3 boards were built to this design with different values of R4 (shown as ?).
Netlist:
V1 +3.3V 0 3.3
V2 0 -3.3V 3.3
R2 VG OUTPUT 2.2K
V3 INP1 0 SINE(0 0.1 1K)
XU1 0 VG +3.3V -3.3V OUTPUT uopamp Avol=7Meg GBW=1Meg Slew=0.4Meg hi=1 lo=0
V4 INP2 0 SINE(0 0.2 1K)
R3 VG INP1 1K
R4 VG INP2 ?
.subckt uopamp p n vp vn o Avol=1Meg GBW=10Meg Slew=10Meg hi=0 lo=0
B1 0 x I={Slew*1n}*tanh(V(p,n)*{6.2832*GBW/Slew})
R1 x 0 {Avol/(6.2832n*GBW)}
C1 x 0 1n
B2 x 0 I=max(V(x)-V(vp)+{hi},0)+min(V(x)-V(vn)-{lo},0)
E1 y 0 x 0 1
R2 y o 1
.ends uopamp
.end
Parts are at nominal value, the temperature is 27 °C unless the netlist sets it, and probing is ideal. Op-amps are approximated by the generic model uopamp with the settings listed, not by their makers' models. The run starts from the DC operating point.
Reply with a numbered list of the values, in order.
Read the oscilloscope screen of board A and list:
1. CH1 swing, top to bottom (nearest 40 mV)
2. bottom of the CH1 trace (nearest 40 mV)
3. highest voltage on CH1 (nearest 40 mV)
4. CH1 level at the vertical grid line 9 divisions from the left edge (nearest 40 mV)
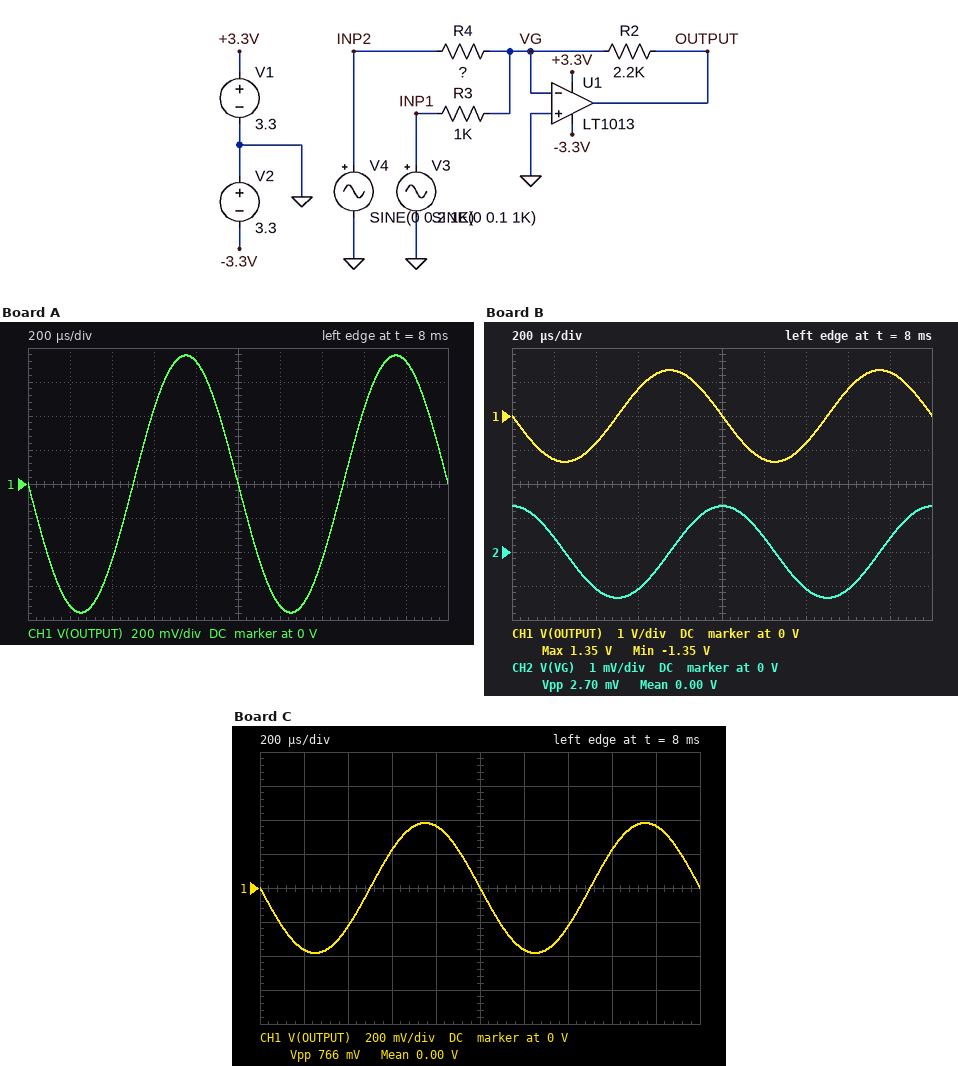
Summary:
1. 1.52 V
2. -760 mV
3. 760 mV
4. 720 mV
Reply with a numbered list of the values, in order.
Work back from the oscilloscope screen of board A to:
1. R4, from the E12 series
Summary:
1. 820 Ω
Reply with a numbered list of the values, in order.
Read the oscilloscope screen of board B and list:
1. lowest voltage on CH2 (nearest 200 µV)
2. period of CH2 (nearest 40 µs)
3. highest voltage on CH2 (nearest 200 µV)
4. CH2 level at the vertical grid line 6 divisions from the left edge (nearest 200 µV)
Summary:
1. -1.4 mV
2. 1.00 ms
3. 1.4 mV
4. 400 µV
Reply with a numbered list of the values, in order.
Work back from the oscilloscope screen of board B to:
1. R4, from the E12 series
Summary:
1. 390 Ω
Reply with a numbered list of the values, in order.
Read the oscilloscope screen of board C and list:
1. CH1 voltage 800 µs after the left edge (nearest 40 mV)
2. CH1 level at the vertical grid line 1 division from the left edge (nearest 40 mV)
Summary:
1. 360 mV
2. -360 mV
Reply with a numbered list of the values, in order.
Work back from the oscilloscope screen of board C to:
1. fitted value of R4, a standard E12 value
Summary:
1. 2.7 kΩ
